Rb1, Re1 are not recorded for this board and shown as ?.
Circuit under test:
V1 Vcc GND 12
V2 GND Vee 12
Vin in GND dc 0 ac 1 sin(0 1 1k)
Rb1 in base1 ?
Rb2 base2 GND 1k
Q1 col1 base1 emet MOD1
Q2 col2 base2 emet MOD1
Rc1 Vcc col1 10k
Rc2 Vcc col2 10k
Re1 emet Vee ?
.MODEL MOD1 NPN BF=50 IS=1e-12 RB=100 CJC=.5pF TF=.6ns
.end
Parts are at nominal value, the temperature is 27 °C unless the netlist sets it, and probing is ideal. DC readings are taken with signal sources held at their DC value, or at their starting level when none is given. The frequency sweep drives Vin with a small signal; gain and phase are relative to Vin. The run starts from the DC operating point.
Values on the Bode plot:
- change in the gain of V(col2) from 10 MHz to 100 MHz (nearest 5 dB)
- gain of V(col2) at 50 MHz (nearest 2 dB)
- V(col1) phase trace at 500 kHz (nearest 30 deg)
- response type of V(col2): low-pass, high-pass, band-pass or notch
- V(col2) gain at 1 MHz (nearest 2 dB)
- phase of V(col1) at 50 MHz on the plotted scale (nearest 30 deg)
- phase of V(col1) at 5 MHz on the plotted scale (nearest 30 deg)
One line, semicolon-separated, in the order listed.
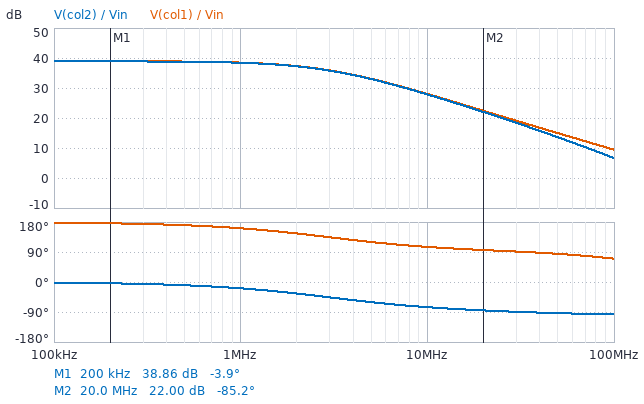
-20 dB; 14 dB; 180 deg; low-pass; 38 dB; 90 deg; 120 deg
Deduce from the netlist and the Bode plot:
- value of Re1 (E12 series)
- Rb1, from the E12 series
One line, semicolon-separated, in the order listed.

8.2 kΩ; 680 Ω
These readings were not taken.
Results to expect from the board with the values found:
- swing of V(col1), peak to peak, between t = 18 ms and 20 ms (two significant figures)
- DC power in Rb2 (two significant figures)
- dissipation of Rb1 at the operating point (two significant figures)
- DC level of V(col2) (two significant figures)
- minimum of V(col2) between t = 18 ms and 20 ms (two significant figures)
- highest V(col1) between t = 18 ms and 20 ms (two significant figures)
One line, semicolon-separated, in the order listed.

12 V; 170 nW; 140 nW; 5.5 V; -610 mV; 12 V
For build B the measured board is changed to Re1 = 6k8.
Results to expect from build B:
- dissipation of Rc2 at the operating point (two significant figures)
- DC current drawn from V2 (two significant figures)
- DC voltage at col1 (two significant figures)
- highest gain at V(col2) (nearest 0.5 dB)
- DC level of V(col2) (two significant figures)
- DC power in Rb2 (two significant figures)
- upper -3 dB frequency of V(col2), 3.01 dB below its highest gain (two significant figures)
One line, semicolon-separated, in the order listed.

6.0 mW; 1.7 mA; 3.2 V; 40.0 dB; 4.3 V; 240 nW; 2.4 MHz
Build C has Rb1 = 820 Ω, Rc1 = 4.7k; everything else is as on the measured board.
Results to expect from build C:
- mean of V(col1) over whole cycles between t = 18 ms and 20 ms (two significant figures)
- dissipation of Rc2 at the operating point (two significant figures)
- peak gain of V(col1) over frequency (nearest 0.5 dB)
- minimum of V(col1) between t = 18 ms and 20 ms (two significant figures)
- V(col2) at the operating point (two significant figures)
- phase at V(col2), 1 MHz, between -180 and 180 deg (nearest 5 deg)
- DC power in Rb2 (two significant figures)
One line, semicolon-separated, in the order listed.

8.6 V; 4.4 mW; 32.0 dB; 5.0 V; 5.4 V; -15 deg; 180 nW
